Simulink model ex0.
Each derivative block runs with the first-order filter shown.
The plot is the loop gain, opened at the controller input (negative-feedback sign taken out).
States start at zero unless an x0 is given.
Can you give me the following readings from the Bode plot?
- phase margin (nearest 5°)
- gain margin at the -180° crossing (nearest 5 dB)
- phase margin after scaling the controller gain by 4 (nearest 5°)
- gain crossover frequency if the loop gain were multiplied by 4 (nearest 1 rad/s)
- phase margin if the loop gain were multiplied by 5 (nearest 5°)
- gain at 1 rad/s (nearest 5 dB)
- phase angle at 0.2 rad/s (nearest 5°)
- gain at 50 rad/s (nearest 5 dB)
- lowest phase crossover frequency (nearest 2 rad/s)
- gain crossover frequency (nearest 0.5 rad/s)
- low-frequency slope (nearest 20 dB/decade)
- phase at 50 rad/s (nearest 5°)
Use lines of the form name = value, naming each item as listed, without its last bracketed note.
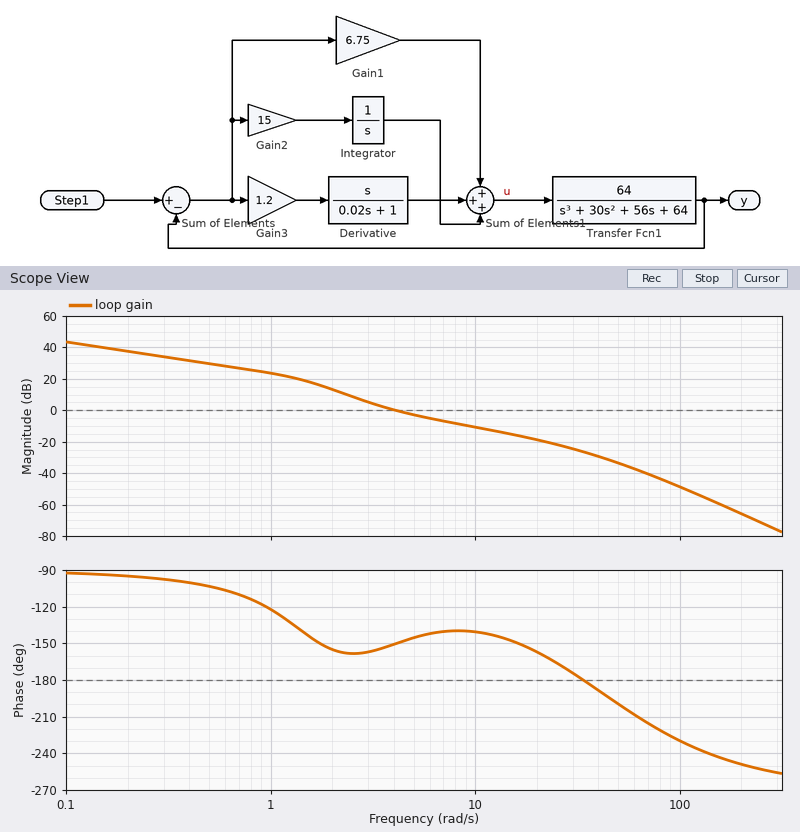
phase margin = 30°
gain margin at the -180° crossing = 25 dB
phase margin after scaling the controller gain by 4 = 40°
gain crossover frequency if the loop gain were multiplied by 4 = 11 rad/s
phase margin if the loop gain were multiplied by 5 = 35°
gain at 1 rad/s = 25 dB
phase angle at 0.2 rad/s = -95°
gain at 50 rad/s = -35 dB
lowest phase crossover frequency = 34 rad/s
gain crossover frequency = 4.0 rad/s
low-frequency slope = -20 dB/decade
phase at 50 rad/s = -200°
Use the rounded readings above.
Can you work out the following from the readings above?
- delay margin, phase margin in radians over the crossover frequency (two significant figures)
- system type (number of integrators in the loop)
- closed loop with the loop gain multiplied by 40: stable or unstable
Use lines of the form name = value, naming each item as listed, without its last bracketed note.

delay margin, phase margin in radians over the crossover frequency = 0.13 s
system type = 1
closed loop with the loop gain multiplied by 40: stable or unstable = unstable
